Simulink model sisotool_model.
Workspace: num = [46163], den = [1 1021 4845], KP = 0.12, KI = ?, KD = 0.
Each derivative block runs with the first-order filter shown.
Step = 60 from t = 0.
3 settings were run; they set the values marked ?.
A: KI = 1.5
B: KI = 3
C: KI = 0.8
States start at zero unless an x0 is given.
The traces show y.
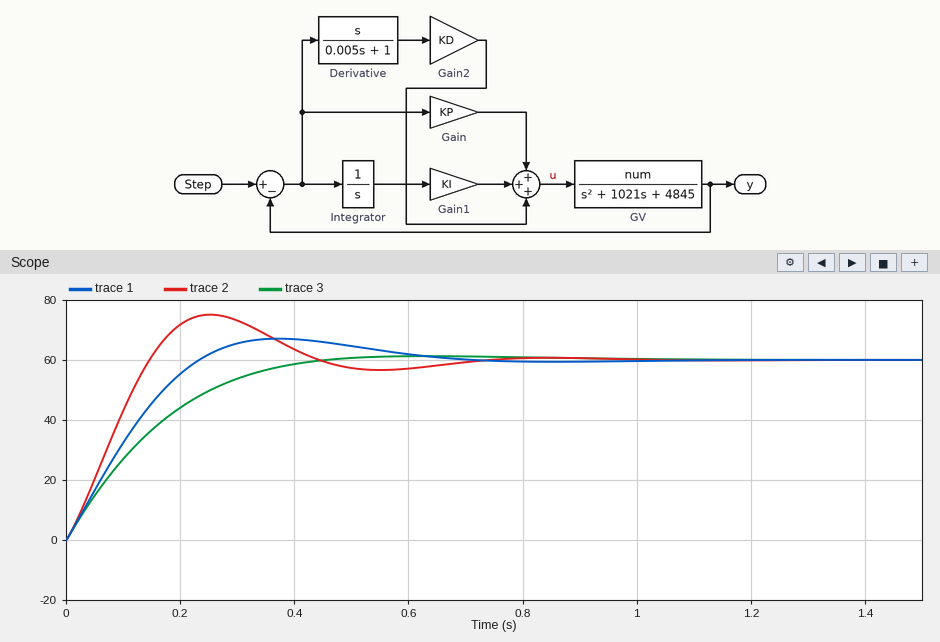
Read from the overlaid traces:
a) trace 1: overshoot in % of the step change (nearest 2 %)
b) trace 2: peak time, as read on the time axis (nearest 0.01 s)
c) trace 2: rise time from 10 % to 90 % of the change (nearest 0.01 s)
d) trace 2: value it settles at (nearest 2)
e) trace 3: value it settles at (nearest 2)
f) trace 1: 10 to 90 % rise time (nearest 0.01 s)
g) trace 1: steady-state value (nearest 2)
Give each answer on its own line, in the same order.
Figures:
12 %
0.25 s
0.11 s
60
60
0.17 s
60
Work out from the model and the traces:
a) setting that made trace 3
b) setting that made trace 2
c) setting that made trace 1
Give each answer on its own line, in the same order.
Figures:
C
B
A
